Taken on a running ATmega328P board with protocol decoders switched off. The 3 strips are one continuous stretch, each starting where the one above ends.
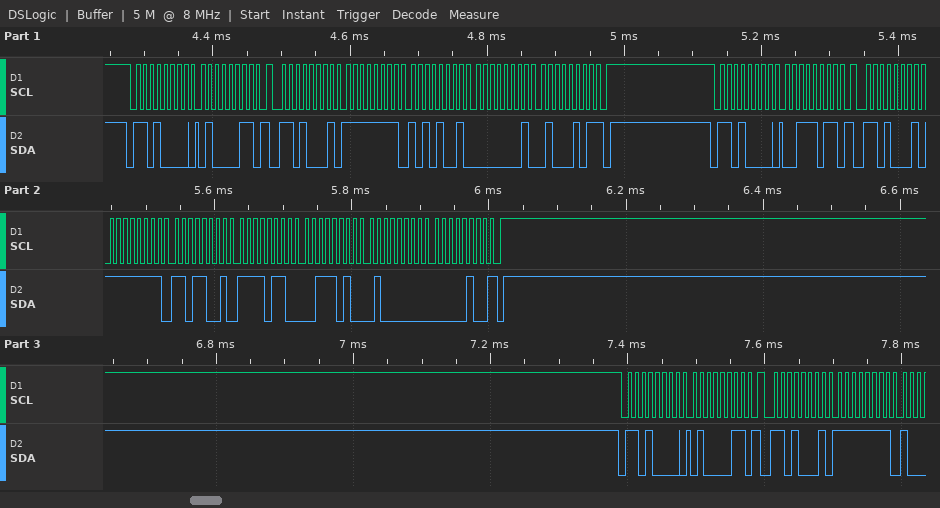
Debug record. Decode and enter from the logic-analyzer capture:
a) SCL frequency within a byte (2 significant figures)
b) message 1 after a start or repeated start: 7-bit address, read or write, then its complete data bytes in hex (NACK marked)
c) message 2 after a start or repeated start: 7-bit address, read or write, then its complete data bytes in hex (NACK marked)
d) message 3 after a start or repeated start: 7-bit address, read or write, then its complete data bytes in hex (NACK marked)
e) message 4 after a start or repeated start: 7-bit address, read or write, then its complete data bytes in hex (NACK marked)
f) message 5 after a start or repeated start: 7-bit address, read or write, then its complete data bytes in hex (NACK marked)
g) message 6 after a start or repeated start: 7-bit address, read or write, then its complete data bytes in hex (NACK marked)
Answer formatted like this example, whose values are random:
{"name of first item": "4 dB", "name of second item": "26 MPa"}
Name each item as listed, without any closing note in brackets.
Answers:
{"SCL frequency within a byte": "100 kHz", "message 1 after a start or repeated start: 7-bit address, read or write, then its complete data bytes in hex": "0x68 write: 43", "message 2 after a start or repeated start: 7-bit address, read or write, then its complete data bytes in hex": "0x68 read: FF A9 01 45 NACK", "message 3 after a start or repeated start: 7-bit address, read or write, then its complete data bytes in hex": "0x68 write: 3B", "message 4 after a start or repeated start: 7-bit address, read or write, then its complete data bytes in hex": "0x68 read: FF D9 F6 3A 40 04 NACK", "message 5 after a start or repeated start: 7-bit address, read or write, then its complete data bytes in hex": "0x68 write: 43", "message 6 after a start or repeated start: 7-bit address, read or write, then its complete data bytes in hex": "0x68 read: FF"}
